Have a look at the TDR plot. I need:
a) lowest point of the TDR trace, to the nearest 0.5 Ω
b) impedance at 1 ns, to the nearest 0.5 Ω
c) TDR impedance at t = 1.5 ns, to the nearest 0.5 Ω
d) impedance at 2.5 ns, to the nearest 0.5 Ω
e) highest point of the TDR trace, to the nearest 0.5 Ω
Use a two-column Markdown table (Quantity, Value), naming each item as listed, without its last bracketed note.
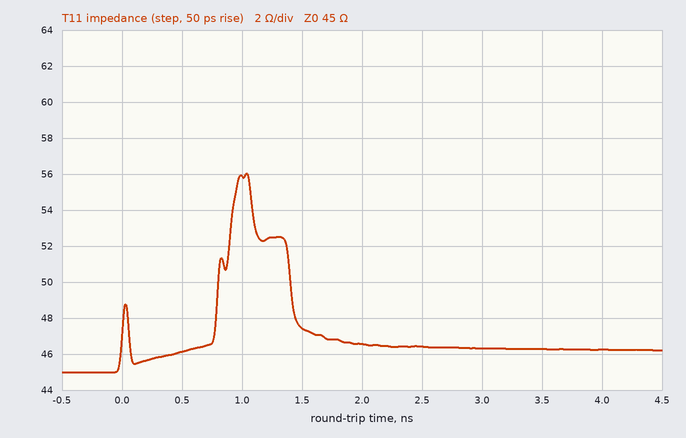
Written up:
| Quantity | Value |
|---|---|
| lowest point of the TDR trace, to the nearest 0.5 Ω | 45.0 Ω |
| impedance at 1 ns, to the nearest 0.5 Ω | 56.0 Ω |
| TDR impedance at t = 1.5 ns, to the nearest 0.5 Ω | 47.5 Ω |
| impedance at 2.5 ns, to the nearest 0.5 Ω | 46.5 Ω |
| highest point of the TDR trace, to the nearest 0.5 Ω | 56.0 Ω |
